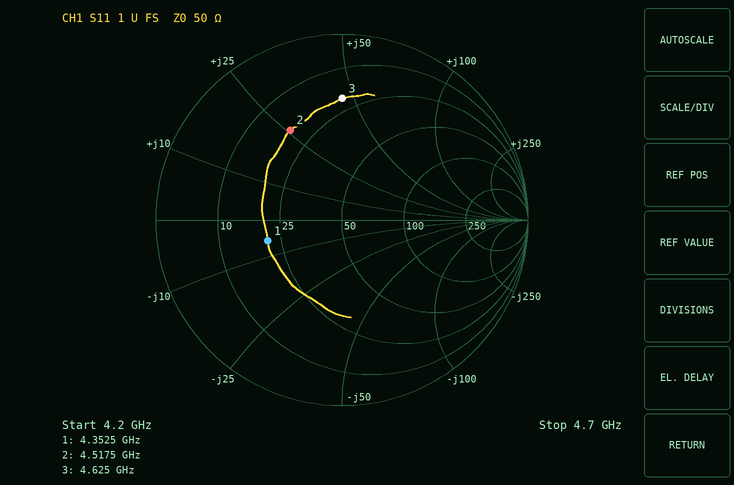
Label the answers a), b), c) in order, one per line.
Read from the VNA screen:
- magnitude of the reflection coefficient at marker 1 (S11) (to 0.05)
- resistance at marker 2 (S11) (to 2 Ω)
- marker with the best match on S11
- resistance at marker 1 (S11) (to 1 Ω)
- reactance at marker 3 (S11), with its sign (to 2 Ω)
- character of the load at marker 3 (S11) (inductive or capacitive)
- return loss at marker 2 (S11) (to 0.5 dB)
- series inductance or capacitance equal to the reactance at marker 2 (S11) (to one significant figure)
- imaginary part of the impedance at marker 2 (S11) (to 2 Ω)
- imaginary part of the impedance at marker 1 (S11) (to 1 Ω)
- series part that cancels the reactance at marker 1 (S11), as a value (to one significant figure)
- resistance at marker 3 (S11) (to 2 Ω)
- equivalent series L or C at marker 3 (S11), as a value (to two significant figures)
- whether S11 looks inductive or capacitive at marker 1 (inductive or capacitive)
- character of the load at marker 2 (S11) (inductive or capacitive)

a) 0.40
b) 18 Ω
c) marker 1
d) 21 Ω
e) +46 Ω
f) inductive
g) 5.0 dB
h) 900 pH
i) +26 Ω
j) -6 Ω
k) 200 pH
l) 20 Ω
m) 1.6 nH
n) capacitive
o) inductive
